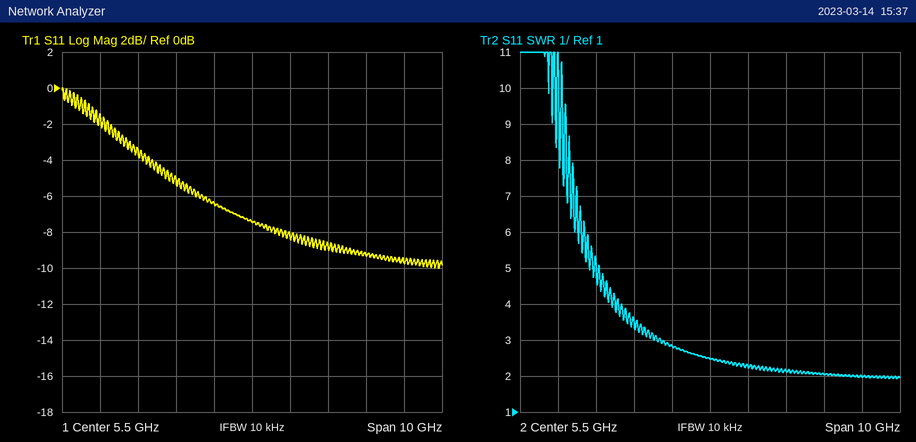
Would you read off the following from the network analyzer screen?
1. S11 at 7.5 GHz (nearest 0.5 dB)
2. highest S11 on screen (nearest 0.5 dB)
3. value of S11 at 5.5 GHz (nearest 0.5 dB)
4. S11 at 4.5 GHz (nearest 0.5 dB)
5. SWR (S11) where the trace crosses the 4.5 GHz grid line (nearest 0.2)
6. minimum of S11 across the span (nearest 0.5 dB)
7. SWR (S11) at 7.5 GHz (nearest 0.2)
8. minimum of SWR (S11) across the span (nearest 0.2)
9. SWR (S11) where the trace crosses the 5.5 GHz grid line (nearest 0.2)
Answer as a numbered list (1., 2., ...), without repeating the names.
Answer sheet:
1. -9.0 dB
2. 0.0 dB
3. -7.5 dB
4. -6.5 dB
5. 2.8
6. -10.0 dB
7. 2.2
8. 2.0
9. 2.4
